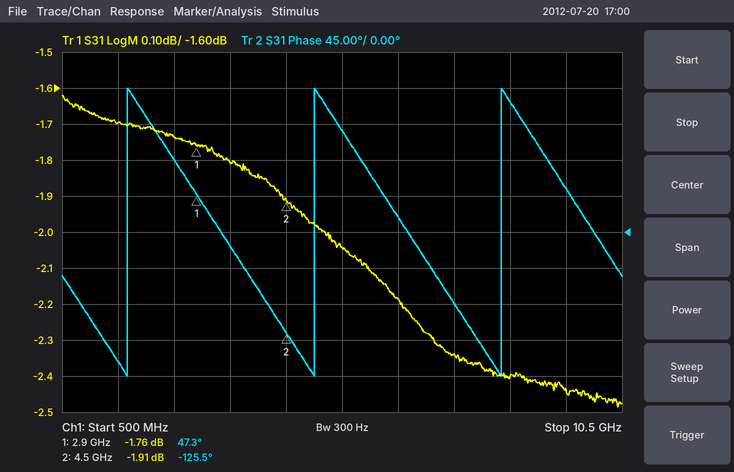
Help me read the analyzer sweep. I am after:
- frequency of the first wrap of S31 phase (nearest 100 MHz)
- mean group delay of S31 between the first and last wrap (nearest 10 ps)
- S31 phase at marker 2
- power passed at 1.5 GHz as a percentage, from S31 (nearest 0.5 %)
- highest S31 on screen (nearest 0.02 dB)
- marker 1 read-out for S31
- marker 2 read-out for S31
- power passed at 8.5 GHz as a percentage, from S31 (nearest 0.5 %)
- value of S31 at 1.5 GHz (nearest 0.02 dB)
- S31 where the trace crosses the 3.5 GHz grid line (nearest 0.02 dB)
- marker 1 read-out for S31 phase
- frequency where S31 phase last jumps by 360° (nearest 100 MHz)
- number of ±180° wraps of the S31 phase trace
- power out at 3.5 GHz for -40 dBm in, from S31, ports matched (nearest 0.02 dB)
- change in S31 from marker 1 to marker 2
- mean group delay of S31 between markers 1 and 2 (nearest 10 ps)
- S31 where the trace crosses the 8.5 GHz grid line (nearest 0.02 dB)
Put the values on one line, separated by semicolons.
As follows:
1.7 GHz; 300 ps; -125.5°; 67.5 %; -1.62 dB; -1.76 dB; -1.91 dB; 57.5 %; -1.70 dB; -1.80 dB; 47.3°; 8.3 GHz; 3; -41.80 dBm; -0.15 dB; 300 ps; -2.40 dB
